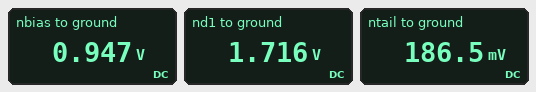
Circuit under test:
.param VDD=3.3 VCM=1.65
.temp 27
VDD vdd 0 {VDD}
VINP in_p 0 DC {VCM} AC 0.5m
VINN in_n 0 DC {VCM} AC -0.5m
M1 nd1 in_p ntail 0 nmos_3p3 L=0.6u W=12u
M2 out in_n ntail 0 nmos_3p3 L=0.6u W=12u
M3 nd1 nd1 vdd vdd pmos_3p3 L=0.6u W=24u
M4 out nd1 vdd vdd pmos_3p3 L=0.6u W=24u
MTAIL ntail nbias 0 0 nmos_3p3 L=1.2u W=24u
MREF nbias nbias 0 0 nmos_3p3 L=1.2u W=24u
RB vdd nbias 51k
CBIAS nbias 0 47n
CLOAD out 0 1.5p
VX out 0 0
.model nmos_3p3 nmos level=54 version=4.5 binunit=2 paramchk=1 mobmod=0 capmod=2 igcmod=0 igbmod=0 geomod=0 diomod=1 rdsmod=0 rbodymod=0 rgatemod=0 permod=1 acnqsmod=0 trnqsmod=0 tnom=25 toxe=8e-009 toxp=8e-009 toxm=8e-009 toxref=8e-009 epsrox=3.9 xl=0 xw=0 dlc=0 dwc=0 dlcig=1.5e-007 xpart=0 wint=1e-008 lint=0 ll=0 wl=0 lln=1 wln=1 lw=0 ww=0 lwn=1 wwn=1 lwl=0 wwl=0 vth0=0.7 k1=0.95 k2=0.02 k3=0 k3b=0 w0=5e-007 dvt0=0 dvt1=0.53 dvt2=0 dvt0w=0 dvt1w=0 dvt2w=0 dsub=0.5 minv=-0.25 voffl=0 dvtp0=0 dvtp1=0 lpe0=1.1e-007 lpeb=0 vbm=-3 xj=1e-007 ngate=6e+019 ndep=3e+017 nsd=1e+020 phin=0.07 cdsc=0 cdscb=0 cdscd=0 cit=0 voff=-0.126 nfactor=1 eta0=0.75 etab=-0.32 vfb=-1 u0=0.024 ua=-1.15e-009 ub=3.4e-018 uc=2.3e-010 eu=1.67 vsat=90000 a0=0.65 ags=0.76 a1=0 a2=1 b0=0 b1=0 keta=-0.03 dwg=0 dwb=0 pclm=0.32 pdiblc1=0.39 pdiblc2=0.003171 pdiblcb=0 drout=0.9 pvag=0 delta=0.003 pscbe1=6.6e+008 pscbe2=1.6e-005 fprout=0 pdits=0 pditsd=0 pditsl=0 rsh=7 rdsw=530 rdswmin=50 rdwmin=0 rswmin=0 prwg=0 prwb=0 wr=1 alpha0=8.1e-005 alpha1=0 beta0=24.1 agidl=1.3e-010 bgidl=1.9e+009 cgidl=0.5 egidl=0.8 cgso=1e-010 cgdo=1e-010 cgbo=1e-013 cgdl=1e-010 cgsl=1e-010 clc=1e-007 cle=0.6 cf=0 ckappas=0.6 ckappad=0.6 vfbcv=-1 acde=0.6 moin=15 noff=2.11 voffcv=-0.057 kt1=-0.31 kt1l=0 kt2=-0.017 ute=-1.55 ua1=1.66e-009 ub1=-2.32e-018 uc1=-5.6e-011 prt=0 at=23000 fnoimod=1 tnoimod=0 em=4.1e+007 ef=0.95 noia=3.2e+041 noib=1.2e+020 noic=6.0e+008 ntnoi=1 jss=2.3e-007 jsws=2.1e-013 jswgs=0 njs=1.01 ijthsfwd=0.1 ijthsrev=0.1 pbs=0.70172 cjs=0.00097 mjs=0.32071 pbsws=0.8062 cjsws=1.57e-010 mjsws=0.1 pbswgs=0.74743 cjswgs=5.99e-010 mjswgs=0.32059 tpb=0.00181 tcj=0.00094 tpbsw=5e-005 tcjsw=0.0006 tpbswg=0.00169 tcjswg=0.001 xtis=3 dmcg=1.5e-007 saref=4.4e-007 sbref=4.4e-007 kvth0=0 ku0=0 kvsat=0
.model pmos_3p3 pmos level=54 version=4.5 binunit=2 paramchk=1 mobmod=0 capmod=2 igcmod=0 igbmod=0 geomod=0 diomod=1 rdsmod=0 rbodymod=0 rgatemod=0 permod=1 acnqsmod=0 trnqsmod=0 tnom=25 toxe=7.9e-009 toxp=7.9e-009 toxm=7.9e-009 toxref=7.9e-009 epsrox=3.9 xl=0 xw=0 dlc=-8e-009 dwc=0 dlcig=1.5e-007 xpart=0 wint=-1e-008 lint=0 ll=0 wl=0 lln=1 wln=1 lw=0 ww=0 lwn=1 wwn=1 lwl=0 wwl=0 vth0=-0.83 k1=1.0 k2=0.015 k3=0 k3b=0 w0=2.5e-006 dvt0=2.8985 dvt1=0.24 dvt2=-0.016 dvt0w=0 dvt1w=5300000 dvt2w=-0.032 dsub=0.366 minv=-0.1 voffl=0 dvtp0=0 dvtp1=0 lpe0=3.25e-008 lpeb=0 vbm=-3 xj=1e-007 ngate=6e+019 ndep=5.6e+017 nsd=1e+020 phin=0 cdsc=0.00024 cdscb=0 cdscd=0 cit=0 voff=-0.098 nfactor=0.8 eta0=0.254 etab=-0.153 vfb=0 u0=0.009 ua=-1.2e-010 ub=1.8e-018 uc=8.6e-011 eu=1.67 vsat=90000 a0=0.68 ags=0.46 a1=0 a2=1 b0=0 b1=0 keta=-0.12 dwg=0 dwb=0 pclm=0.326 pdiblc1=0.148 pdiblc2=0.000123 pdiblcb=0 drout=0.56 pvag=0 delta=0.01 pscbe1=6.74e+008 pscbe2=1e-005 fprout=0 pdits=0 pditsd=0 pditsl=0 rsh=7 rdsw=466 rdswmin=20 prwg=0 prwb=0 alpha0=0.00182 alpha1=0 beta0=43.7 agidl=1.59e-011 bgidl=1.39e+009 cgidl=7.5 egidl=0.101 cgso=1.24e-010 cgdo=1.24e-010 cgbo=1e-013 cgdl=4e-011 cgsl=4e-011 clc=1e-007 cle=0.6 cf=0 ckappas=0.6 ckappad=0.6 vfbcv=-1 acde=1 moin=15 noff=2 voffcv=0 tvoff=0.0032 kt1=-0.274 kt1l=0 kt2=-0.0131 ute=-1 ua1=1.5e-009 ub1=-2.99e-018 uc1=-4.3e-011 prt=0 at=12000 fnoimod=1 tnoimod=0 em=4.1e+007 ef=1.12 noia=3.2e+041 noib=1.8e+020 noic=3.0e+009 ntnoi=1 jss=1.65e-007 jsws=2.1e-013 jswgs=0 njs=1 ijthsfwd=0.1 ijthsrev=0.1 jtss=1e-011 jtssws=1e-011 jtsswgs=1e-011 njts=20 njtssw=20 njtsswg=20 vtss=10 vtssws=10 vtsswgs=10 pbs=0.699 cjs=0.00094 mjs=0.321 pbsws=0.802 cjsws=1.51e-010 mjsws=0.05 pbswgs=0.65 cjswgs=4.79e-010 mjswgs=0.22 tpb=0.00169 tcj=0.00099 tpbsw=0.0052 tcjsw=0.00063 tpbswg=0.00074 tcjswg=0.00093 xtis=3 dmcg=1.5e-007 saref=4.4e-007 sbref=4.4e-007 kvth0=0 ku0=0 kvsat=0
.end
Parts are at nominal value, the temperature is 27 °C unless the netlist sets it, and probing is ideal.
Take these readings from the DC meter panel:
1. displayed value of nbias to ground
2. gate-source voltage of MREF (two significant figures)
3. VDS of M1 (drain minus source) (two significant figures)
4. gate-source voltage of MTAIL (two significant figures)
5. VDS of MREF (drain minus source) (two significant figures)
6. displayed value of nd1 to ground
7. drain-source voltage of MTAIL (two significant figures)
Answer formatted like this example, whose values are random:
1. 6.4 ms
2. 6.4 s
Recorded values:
1. 0.947 V
2. 950 mV
3. 1.5 V
4. 950 mV
5. 950 mV
6. 1.716 V
7. 190 mV
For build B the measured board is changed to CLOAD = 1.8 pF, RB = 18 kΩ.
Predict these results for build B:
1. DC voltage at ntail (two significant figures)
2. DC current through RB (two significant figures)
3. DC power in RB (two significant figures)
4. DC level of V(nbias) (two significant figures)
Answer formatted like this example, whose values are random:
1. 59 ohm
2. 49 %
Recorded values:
1. 170 mV
2. 120 µA
3. 270 µW
4. 1.1 V
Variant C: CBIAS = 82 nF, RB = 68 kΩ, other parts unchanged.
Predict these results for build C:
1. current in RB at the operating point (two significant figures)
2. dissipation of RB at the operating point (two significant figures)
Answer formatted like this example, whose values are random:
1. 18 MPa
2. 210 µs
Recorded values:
1. 35 µA
2. 84 µW
